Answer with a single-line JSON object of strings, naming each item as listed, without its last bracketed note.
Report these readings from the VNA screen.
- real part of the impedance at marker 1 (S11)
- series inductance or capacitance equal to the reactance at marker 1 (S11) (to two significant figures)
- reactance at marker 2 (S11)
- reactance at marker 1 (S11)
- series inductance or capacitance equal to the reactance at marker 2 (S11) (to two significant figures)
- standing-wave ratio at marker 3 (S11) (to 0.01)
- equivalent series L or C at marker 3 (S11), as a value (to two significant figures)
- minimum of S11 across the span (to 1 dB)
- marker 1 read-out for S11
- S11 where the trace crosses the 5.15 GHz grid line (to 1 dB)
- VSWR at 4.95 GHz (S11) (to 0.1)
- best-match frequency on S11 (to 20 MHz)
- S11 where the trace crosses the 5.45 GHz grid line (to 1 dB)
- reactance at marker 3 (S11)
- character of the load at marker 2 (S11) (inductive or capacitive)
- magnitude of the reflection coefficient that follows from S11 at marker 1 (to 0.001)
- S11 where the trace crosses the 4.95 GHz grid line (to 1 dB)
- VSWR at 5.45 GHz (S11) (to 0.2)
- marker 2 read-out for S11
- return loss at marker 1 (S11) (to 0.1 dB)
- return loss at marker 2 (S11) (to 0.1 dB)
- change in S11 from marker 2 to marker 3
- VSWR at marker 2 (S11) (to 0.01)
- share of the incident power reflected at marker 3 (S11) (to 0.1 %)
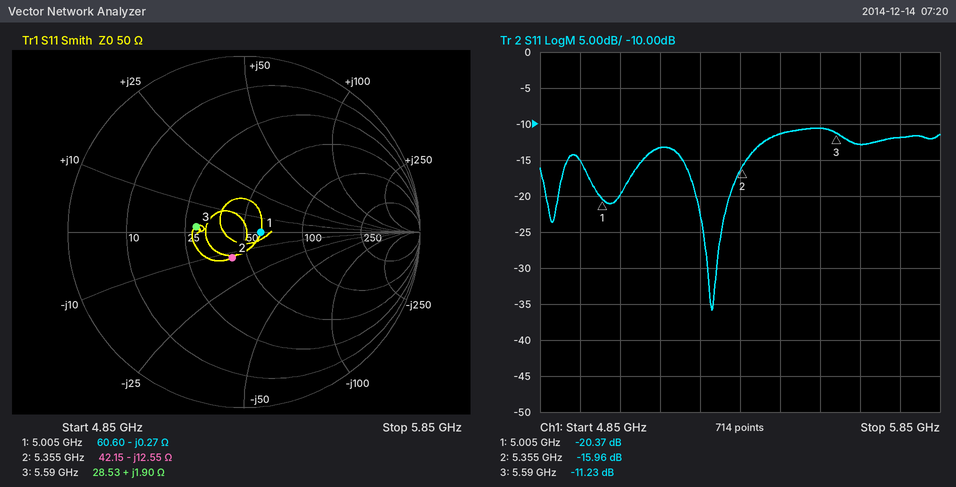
{"real part of the impedance at marker 1": "60.60 Ω", "series inductance or capacitance equal to the reactance at marker 1 (S11)": "120 pF", "reactance at marker 2": "-12.55 Ω", "reactance at marker 1": "-0.27 Ω", "series inductance or capacitance equal to the reactance at marker 2 (S11)": "2.4 pF", "standing-wave ratio at marker 3 (S11)": "1.76", "equivalent series L or C at marker 3 (S11), as a value": "54 pH", "minimum of S11 across the span": "-36 dB", "marker 1 read-out for S11": "-20.37 dB", "S11 where the trace crosses the 5.15 GHz grid line": "-13 dB", "VSWR at 4.95 GHz (S11)": "1.4", "best-match frequency on S11": "5.28 GHz", "S11 where the trace crosses the 5.45 GHz grid line": "-11 dB", "reactance at marker 3": "+1.90 Ω", "character of the load at marker 2 (S11)": "capacitive", "magnitude of the reflection coefficient that follows from S11 at marker 1": "0.096", "S11 where the trace crosses the 4.95 GHz grid line": "-15 dB", "VSWR at 5.45 GHz (S11)": "1.8", "marker 2 read-out for S11": "-15.96 dB", "return loss at marker 1 (S11)": "20.4 dB", "return loss at marker 2 (S11)": "16.0 dB", "change in S11 from marker 2 to marker 3": "4.73 dB", "VSWR at marker 2 (S11)": "1.38", "share of the incident power reflected at marker 3 (S11)": "7.5 %"}
